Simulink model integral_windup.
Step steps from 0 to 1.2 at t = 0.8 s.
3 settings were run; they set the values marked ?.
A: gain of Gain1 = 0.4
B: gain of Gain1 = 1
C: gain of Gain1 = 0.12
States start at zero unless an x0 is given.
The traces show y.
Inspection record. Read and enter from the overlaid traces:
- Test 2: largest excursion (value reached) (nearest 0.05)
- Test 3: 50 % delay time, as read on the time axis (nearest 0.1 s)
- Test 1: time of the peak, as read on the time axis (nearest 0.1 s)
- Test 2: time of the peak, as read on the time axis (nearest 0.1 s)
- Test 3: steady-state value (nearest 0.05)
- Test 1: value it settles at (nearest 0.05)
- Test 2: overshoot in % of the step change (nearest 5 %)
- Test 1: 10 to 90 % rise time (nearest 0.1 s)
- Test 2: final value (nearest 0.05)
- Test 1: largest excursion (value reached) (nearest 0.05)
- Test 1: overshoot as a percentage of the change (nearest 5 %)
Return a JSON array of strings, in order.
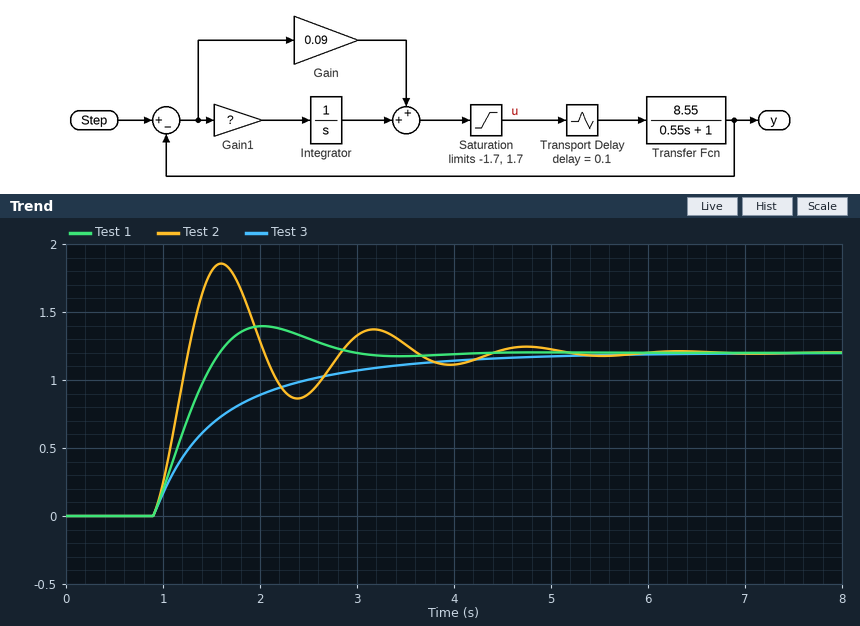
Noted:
["1.85", "1.4 s", "2.0 s", "1.6 s", "1.20", "1.20", "55 %", "0.5 s", "1.20", "1.40", "15 %"]
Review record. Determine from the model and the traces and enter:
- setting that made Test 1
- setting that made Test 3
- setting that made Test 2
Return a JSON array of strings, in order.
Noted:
["A", "C", "B"]
